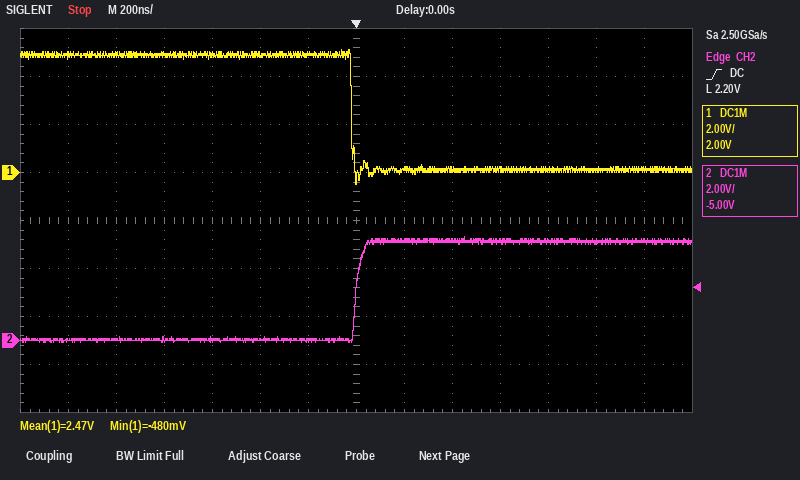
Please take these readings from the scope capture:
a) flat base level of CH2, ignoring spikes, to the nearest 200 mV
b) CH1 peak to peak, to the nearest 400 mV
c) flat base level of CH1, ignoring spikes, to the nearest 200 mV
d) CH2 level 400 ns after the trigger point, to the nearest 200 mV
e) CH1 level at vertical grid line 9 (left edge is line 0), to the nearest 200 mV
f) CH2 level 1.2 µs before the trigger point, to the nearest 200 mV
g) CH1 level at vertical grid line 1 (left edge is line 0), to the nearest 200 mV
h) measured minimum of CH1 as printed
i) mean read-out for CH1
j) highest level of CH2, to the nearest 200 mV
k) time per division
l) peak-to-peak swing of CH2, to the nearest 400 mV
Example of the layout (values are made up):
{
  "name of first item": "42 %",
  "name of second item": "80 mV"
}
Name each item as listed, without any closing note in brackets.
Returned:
{
  "flat base level of CH2, ignoring spikes, to the nearest 200 mV": "0.0 V",
  "CH1 peak to peak, to the nearest 400 mV": "5.6 V",
  "flat base level of CH1, ignoring spikes, to the nearest 200 mV": "200 mV",
  "CH2 level 400 ns after the trigger point, to the nearest 200 mV": "4.2 V",
  "CH1 level at vertical grid line 9 (left edge is line 0), to the nearest 200 mV": "200 mV",
  "CH2 level 1.2 µs before the trigger point, to the nearest 200 mV": "0.0 V",
  "CH1 level at vertical grid line 1 (left edge is line 0), to the nearest 200 mV": "4.8 V",
  "measured minimum of CH1 as printed": "-480 mV",
  "mean read-out for CH1": "2.47 V",
  "highest level of CH2, to the nearest 200 mV": "4.4 V",
  "time per division": "200 ns",
  "peak-to-peak swing of CH2, to the nearest 400 mV": "4.4 V"
}
